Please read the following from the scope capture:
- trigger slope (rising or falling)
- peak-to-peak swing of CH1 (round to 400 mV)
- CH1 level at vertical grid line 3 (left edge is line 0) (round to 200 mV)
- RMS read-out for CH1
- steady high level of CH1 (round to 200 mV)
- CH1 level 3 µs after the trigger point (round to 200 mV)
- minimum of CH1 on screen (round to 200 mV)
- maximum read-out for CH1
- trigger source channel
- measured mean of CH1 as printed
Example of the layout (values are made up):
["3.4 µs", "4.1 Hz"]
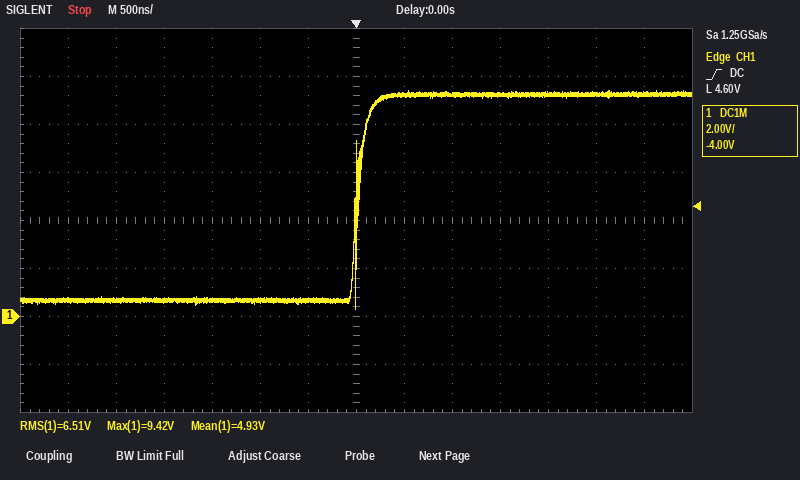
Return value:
["rising", "9.2 V", "600 mV", "6.51 V", "9.2 V", "9.2 V", "400 mV", "9.42 V", "CH1", "4.93 V"]
